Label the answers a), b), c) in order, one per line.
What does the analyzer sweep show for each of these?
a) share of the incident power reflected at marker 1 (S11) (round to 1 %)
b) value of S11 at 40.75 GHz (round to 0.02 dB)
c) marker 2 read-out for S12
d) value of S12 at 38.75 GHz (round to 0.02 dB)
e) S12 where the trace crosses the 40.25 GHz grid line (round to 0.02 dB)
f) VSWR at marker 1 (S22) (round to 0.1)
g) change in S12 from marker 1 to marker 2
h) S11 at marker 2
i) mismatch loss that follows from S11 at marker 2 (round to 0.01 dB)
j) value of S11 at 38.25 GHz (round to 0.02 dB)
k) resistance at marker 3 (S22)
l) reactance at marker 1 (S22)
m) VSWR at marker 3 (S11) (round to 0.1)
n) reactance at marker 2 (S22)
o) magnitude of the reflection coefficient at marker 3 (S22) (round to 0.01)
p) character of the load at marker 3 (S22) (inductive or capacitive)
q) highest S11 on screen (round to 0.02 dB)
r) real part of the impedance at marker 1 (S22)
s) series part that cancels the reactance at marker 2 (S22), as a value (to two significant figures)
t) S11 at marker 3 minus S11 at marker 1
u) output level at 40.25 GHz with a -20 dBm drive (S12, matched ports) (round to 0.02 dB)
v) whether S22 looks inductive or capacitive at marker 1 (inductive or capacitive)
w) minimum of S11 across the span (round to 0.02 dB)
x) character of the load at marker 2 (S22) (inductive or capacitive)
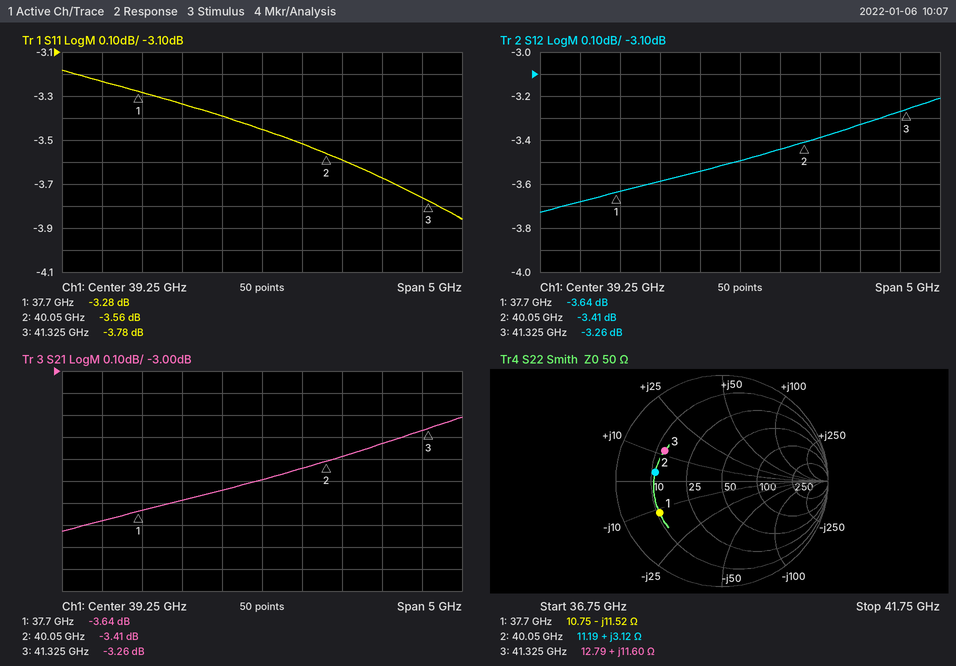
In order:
a) 47 %
b) -3.68 dB
c) -3.41 dB
d) -3.54 dB
e) -3.38 dB
f) 4.9
g) 0.23 dB
h) -3.56 dB
i) 2.52 dB
j) -3.34 dB
k) 12.79 Ω
l) -11.52 Ω
m) 4.7
n) +3.12 Ω
o) 0.61
p) inductive
q) -3.18 dB
r) 10.75 Ω
s) 1.3 pF
t) -0.50 dB
u) -23.38 dBm
v) capacitive
w) -3.86 dB
x) inductive
